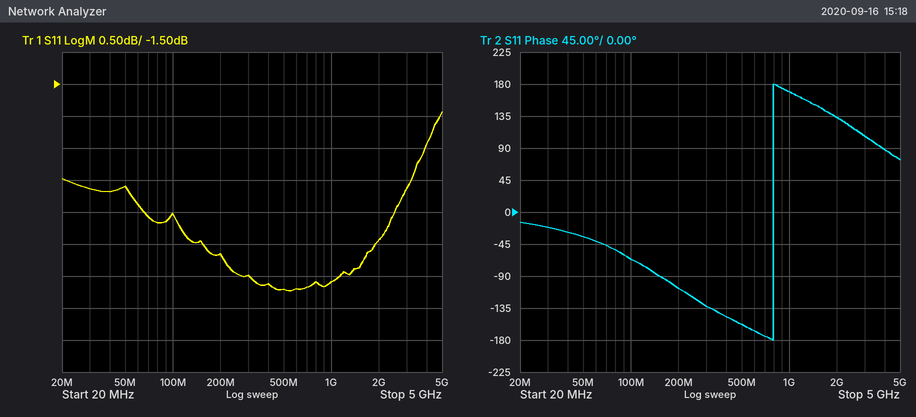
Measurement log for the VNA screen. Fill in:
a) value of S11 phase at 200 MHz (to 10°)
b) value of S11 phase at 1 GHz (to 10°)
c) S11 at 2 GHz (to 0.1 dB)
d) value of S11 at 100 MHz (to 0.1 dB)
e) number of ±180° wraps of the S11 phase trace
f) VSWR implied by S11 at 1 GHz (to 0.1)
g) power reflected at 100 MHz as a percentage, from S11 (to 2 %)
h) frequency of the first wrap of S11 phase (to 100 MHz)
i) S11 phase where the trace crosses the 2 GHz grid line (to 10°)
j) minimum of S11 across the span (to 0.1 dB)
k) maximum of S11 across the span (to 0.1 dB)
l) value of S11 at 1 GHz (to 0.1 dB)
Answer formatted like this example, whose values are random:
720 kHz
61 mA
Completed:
-110°
170°
-3.9 dB
-3.5 dB
1
3.9
44 %
800 MHz
130°
-4.7 dB
-1.9 dB
-4.6 dB
